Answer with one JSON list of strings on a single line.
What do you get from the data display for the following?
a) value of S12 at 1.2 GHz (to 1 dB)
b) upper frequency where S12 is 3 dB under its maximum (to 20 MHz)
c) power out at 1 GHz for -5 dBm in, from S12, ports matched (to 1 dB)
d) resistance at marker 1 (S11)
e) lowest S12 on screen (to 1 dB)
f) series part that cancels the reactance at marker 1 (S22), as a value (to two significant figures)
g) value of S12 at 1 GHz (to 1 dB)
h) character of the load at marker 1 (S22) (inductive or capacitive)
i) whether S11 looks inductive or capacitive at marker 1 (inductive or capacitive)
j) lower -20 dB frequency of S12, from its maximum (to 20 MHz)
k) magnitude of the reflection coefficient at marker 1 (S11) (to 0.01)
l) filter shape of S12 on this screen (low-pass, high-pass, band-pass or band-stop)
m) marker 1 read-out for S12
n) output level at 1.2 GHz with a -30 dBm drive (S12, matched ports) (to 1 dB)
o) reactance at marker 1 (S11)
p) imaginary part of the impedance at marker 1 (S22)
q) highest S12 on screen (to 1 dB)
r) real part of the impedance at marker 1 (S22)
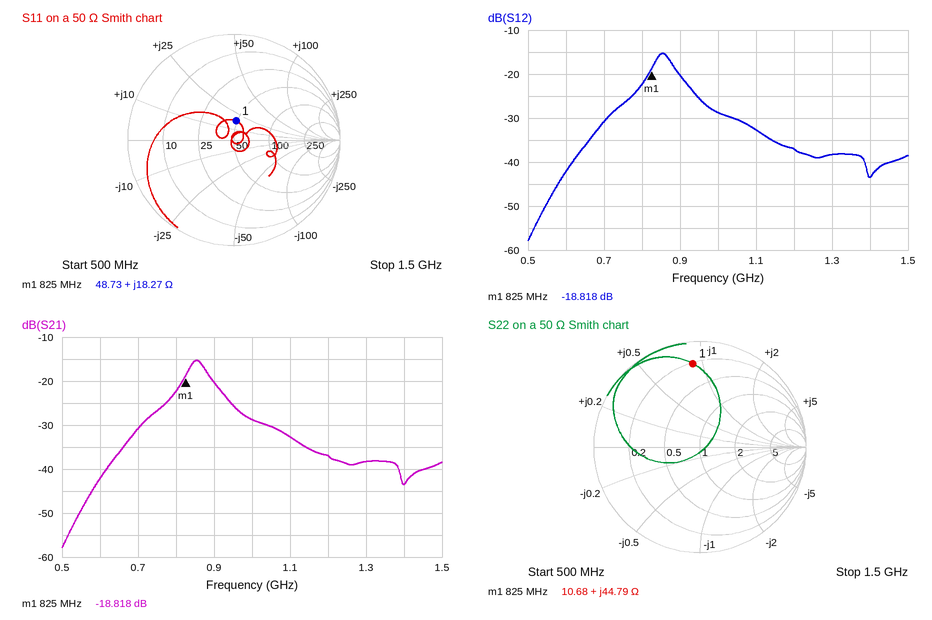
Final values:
["-37 dB", "880 MHz", "-34 dBm", "48.73 Ω", "-58 dB", "4.3 pF", "-29 dB", "inductive", "inductive", "660 MHz", "0.18", "band-pass", "-18.818 dB", "-67 dBm", "+18.27 Ω", "+44.79 Ω", "-15 dB", "10.68 Ω"]
